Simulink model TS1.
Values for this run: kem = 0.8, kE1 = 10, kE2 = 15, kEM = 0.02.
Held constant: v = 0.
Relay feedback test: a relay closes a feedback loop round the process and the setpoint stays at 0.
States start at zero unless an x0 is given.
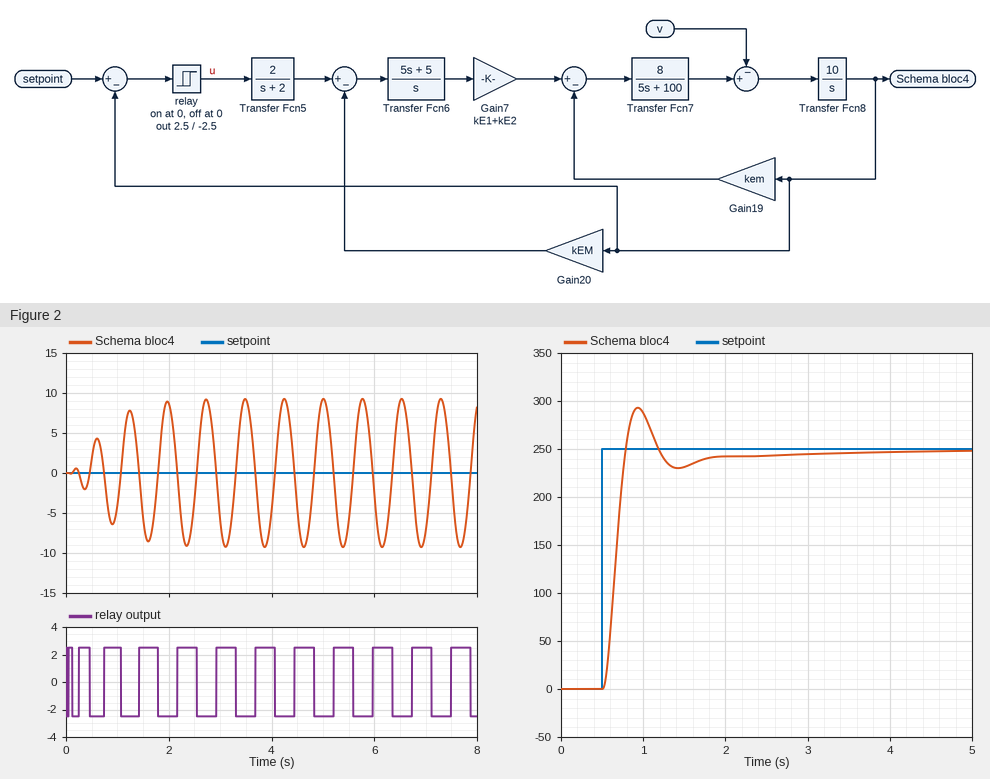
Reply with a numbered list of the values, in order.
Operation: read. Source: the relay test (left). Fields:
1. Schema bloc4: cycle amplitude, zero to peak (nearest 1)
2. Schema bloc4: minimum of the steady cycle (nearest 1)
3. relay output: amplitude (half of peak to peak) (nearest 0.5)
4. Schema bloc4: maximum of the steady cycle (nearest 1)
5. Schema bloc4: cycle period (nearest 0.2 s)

1. 9
2. -9
3. 2.5
4. 9
5. 0.8 s
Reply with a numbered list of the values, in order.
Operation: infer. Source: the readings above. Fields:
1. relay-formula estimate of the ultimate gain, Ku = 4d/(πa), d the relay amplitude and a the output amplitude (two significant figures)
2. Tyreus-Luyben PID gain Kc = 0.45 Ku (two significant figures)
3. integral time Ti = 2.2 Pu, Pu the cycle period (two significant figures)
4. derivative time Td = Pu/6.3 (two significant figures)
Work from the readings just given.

1. 0.35
2. 0.16
3. 1.8 s
4. 0.13 s
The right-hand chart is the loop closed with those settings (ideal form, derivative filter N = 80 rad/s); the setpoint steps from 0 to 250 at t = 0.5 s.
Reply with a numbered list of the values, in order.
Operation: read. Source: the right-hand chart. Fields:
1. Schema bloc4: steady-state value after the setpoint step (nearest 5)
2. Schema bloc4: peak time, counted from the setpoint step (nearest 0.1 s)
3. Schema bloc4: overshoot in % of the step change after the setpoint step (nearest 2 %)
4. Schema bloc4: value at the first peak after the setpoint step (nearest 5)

1. 250
2. 0.4 s
3. 18 %
4. 295
